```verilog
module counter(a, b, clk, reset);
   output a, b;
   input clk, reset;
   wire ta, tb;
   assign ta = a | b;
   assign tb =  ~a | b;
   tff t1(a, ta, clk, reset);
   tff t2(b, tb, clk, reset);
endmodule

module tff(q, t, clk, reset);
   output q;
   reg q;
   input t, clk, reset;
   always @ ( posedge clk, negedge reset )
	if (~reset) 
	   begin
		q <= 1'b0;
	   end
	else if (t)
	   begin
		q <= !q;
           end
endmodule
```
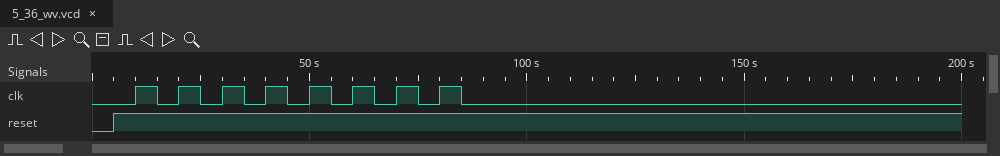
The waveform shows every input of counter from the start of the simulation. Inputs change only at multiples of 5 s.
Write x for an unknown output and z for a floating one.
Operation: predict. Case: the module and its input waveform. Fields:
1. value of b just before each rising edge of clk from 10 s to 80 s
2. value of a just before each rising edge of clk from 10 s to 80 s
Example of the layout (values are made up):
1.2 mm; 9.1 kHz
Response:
0 1 0 0 1 0 0 1; 0 0 1 0 0 1 0 0
